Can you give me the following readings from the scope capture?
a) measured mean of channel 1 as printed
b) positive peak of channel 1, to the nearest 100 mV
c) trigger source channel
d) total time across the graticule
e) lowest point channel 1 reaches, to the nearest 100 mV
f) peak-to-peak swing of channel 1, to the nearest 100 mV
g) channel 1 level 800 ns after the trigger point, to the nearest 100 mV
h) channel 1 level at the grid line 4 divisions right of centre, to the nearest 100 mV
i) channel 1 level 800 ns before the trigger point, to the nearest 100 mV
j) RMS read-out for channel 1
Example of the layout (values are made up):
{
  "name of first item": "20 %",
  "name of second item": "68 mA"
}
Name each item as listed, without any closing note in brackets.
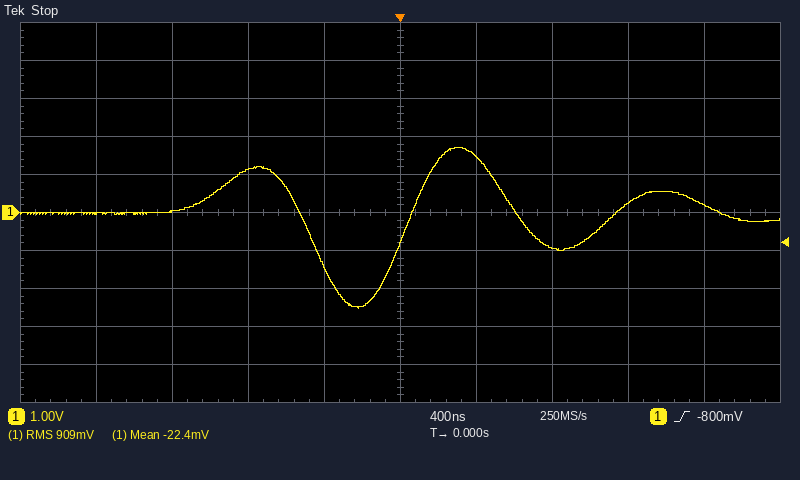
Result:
{
  "measured mean of channel 1 as printed": "-22.4 mV",
  "positive peak of channel 1, to the nearest 100 mV": "1.7 V",
  "trigger source channel": "channel 1",
  "total time across the graticule": "4 µs",
  "lowest point channel 1 reaches, to the nearest 100 mV": "-2.5 V",
  "peak-to-peak swing of channel 1, to the nearest 100 mV": "4.2 V",
  "channel 1 level 800 ns after the trigger point, to the nearest 100 mV": "-900 mV",
  "channel 1 level at the grid line 4 divisions right of centre, to the nearest 100 mV": "200 mV",
  "channel 1 level 800 ns before the trigger point, to the nearest 100 mV": "1.1 V",
  "RMS read-out for channel 1": "909 mV"
}
